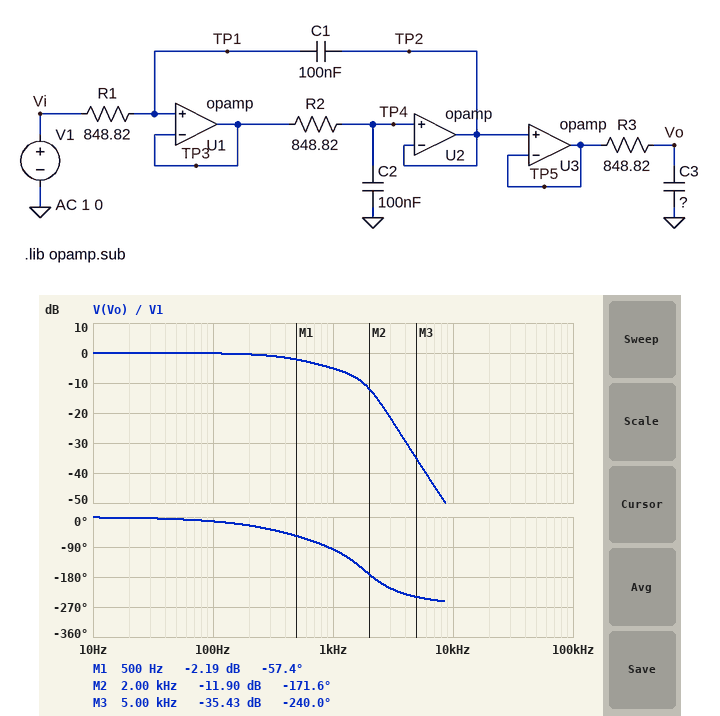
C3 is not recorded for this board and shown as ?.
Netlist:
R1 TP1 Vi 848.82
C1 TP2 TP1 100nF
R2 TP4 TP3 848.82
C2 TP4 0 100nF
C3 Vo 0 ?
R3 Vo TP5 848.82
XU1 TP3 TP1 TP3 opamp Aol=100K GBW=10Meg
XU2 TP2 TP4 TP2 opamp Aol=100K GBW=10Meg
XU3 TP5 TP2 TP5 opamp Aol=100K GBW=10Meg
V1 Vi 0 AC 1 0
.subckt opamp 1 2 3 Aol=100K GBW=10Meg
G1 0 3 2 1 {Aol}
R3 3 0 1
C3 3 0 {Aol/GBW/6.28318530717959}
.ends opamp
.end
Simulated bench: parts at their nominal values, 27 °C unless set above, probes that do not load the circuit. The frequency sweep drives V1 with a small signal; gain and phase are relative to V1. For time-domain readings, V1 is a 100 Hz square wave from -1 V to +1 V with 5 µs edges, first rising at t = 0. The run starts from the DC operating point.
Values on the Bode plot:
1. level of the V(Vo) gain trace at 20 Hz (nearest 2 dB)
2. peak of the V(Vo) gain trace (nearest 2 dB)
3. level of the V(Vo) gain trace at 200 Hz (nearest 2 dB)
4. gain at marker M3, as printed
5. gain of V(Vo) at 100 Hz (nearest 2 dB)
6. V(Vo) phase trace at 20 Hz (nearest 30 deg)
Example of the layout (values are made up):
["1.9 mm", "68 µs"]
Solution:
["0 dB", "0 dB", "0 dB", "-35.43 dB", "0 dB", "0 deg"]
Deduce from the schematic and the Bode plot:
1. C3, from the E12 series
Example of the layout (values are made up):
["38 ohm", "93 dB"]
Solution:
["330 nF"]
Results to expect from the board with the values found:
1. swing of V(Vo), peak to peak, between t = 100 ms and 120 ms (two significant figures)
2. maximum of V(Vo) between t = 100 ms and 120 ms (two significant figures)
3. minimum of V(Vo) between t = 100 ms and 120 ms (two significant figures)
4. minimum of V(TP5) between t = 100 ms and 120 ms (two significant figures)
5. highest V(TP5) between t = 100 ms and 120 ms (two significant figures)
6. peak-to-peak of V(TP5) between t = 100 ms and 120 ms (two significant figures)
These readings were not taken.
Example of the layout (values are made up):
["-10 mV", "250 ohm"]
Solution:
["2.0 V", "1.0 V", "-1.0 V", "-1.3 V", "1.3 V", "2.7 V"]
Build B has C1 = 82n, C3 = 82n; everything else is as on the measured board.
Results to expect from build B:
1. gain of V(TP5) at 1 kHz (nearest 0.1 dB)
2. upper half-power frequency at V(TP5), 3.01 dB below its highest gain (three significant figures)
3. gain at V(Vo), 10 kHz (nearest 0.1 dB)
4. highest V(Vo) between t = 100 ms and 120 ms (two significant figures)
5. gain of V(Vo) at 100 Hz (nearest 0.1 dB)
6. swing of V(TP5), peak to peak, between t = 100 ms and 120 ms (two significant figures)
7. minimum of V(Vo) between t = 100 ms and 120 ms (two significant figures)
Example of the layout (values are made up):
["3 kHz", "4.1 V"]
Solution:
["0.6 dB", "2.37 kHz", "-40.3 dB", "1.1 V", "0 dB", "2.5 V", "-1.1 V"]
